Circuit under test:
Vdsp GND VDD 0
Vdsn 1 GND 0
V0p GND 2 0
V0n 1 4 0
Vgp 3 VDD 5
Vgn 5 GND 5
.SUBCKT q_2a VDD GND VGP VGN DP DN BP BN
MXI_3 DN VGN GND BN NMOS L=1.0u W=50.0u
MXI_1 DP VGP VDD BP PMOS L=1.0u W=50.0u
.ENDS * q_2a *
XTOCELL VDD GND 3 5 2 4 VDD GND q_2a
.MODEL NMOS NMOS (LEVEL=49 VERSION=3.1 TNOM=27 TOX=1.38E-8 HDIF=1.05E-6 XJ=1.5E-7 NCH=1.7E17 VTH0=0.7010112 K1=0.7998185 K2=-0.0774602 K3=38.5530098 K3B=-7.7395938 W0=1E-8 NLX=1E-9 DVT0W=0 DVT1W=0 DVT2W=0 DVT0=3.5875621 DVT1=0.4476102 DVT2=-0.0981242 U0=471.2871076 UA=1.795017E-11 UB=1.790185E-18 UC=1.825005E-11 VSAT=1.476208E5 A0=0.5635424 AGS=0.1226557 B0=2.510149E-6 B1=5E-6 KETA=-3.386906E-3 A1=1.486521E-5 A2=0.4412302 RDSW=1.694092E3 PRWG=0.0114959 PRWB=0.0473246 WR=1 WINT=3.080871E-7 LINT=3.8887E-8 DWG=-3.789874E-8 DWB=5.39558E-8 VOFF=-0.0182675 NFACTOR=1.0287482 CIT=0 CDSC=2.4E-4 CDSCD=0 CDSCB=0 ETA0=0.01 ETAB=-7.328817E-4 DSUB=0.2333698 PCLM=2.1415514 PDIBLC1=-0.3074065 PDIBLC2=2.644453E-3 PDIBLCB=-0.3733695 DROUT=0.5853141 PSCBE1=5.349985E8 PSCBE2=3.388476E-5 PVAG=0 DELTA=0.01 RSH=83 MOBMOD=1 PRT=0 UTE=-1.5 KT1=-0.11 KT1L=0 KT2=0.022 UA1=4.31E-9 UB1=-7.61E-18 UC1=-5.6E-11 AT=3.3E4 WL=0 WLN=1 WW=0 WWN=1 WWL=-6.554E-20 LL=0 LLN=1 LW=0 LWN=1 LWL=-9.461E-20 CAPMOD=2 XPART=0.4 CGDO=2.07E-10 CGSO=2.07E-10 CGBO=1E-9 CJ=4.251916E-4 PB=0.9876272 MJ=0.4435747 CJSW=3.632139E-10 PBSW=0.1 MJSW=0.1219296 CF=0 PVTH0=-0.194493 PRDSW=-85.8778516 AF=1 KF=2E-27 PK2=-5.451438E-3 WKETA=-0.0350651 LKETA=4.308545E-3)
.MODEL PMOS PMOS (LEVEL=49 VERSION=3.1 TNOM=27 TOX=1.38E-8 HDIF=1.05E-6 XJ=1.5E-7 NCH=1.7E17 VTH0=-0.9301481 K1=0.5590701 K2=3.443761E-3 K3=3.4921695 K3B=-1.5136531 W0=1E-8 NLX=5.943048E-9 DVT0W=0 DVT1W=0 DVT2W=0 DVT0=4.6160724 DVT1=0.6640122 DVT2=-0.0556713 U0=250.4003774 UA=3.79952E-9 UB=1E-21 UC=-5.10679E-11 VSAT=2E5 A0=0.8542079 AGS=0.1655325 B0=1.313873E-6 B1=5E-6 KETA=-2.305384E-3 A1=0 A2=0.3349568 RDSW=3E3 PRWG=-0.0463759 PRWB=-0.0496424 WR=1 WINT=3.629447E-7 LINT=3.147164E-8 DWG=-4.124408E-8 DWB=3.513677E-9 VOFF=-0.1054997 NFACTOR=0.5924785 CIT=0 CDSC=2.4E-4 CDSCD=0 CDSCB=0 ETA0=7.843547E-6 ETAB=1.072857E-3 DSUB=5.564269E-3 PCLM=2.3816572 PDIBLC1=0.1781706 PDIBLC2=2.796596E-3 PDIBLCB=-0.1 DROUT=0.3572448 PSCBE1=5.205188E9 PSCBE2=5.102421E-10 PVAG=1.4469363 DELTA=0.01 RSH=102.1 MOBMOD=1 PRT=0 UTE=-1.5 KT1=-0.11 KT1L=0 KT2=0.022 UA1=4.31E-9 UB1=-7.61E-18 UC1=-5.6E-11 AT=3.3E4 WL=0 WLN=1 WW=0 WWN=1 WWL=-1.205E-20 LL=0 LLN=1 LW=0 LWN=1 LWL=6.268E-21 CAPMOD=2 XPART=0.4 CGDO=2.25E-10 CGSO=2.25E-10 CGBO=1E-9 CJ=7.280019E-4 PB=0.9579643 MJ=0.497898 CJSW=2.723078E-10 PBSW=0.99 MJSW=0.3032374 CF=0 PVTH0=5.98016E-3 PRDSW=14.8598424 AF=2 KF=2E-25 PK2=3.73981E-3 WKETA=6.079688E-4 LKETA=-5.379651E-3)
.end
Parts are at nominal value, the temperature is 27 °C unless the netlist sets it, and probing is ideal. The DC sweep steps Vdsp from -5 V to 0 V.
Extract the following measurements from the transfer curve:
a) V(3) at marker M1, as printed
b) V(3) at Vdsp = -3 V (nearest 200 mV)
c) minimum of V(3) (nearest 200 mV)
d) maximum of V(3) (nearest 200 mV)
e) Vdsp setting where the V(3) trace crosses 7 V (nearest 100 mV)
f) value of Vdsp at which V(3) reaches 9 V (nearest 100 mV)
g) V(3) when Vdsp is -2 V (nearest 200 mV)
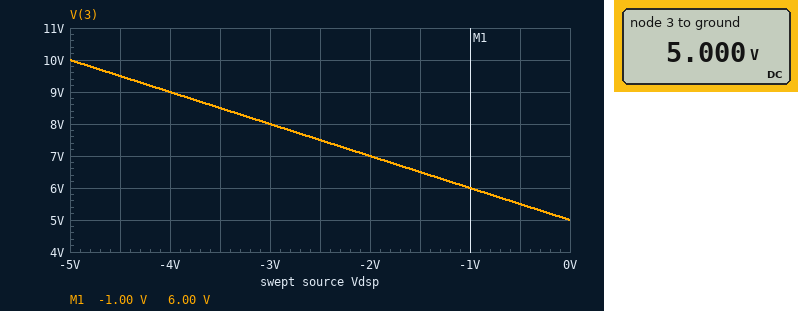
6.00 V
8.0 V
5.0 V
10.0 V
-2.0 V
-4.0 V
7.0 V
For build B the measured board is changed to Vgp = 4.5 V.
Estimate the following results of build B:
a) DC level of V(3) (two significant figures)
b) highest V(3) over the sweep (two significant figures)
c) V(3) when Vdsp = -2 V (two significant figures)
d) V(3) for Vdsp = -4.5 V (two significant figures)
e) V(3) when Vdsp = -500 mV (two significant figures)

4.5 V
9.5 V
6.5 V
9.0 V
5.0 V
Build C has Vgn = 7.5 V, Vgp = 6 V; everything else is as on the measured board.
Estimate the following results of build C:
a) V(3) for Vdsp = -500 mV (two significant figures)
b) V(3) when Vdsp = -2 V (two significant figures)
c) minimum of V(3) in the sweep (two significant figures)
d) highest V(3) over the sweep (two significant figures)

6.5 V
8.0 V
6.0 V
11 V
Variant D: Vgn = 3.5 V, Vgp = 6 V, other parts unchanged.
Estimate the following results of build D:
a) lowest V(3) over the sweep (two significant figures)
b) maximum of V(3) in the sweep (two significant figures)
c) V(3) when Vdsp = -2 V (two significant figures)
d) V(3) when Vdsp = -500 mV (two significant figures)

6.0 V
11 V
8.0 V
6.5 V
